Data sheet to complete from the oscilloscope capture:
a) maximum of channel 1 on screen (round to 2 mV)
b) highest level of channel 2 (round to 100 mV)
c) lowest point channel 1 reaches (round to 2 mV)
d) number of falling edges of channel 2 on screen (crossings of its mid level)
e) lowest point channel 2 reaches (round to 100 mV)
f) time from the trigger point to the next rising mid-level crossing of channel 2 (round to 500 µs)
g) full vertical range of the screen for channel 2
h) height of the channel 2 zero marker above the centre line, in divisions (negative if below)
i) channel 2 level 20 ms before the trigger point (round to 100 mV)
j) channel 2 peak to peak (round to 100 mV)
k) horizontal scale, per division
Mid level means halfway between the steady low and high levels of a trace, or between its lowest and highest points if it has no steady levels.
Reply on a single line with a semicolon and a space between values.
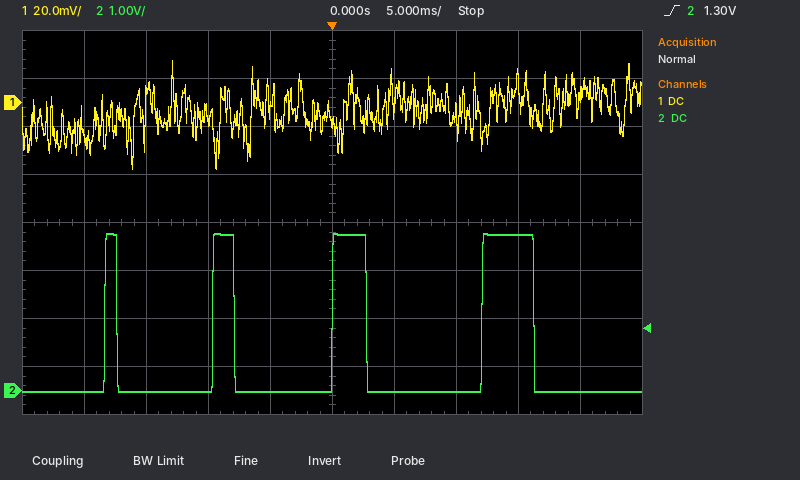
18 mV; 3.3 V; -28 mV; 4; 0.0 V; 12.0 ms; 8 V; -3.5 div; 0.0 V; 3.3 V; 5 ms
